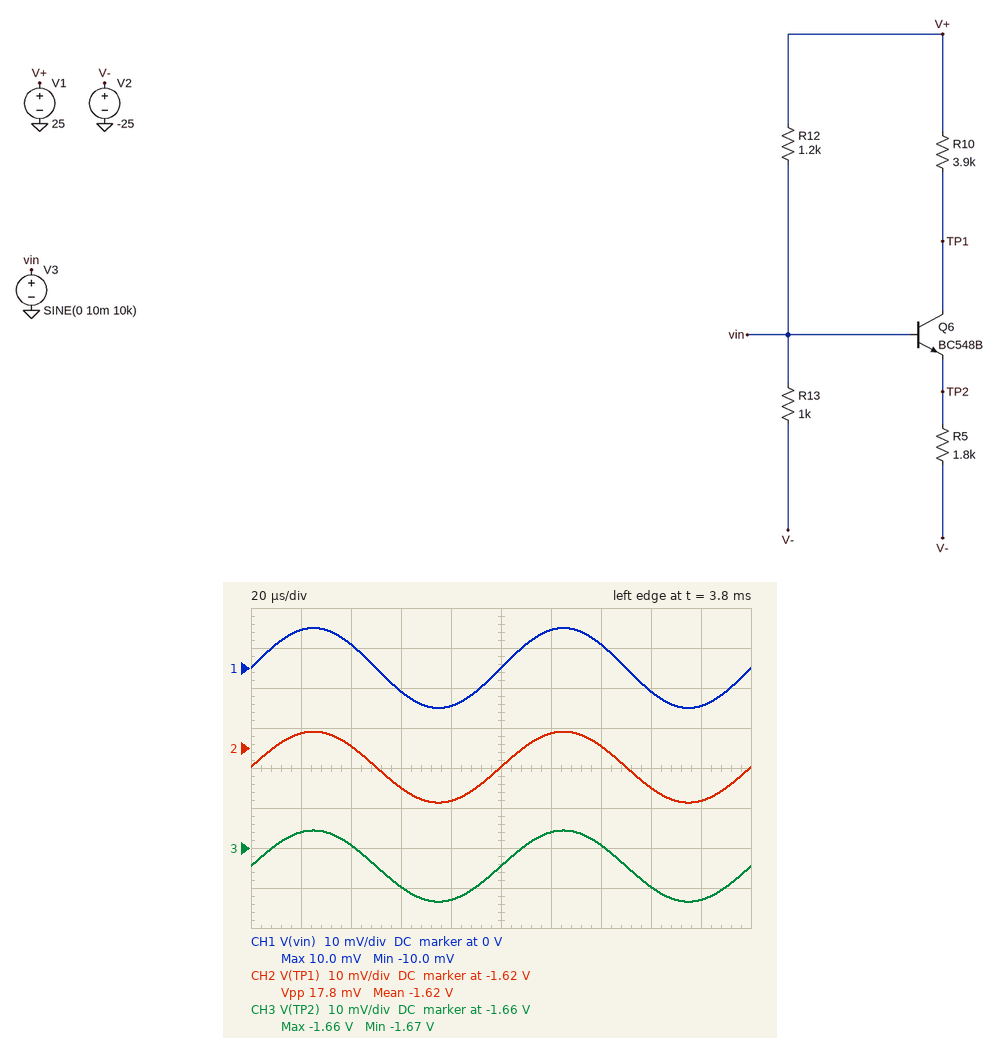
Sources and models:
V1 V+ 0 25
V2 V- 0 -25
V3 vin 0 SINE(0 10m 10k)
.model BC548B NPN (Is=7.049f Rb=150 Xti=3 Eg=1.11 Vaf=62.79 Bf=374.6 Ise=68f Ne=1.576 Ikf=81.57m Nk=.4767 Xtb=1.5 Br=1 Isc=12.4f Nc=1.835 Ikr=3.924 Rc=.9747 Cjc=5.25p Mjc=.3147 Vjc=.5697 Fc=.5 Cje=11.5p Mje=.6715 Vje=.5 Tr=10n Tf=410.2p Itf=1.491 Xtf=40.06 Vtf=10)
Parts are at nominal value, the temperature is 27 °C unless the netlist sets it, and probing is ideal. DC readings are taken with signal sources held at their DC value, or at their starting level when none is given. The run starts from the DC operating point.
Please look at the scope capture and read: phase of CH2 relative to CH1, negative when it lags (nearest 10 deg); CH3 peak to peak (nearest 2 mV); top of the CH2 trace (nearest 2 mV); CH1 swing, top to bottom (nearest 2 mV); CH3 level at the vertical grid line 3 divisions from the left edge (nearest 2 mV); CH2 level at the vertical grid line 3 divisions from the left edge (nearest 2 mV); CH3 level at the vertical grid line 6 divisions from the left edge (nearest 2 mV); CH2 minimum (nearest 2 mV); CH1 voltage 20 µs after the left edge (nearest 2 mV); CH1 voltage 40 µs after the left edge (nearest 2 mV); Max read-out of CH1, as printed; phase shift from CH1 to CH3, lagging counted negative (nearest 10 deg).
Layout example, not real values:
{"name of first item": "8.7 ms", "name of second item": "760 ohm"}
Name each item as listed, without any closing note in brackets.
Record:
{"phase of CH2 relative to CH1, negative when it lags": "0 deg", "CH3 peak to peak": "18 mV", "top of the CH2 trace": "-1.616 V", "CH1 swing, top to bottom": "20 mV", "CH3 level at the vertical grid line 3 divisions from the left edge": "-1.670 V", "CH2 level at the vertical grid line 3 divisions from the left edge": "-1.630 V", "CH3 level at the vertical grid line 6 divisions from the left edge": "-1.656 V", "CH2 minimum": "-1.634 V", "CH1 voltage 20 µs after the left edge": "10 mV", "CH1 voltage 40 µs after the left edge": "6 mV", "Max read-out of CH1, as printed": "10.0 mV", "phase shift from CH1 to CH3, lagging counted negative": "0 deg"}
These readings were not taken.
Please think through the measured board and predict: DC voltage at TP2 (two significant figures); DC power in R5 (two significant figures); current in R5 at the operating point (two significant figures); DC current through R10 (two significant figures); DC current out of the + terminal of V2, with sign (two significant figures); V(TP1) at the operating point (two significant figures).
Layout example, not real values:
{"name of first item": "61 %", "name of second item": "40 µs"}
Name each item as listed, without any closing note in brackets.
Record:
{"DC voltage at TP2": "-1.7 V", "DC power in R5": "300 mW", "current in R5 at the operating point": "13 mA", "DC current through R10": "6.8 mA", "DC current out of the + terminal of V2, with sign": "-38 mA", "V(TP1) at the operating point": "-1.6 V"}
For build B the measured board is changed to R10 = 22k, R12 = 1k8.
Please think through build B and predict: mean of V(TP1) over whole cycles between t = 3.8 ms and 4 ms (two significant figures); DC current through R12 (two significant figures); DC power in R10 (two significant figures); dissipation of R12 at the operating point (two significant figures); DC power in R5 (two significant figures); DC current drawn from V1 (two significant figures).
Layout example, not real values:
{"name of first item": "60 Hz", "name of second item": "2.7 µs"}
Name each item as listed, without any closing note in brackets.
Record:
{"mean of V(TP1) over whole cycles between t = 3.8 ms and 4 ms": "-2.4 V", "DC current through R12": "14 mA", "DC power in R10": "34 mW", "dissipation of R12 at the operating point": "350 mW", "DC power in R5": "280 mW", "DC current drawn from V1": "15 mA"}
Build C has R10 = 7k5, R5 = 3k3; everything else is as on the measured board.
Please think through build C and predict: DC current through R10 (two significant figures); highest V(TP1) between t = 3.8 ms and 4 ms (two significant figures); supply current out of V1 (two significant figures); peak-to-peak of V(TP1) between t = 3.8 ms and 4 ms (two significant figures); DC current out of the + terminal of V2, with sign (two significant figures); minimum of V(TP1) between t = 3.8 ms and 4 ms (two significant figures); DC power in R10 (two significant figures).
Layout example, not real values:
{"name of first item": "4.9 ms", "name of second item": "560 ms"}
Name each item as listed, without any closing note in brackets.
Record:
{"DC current through R10": "3.5 mA", "highest V(TP1) between t = 3.8 ms and 4 ms": "-1.2 V", "supply current out of V1": "24 mA", "peak-to-peak of V(TP1) between t = 3.8 ms and 4 ms": "19 mV", "DC current out of the + terminal of V2, with sign": "-32 mA", "minimum of V(TP1) between t = 3.8 ms and 4 ms": "-1.3 V", "DC power in R10": "92 mW"}
